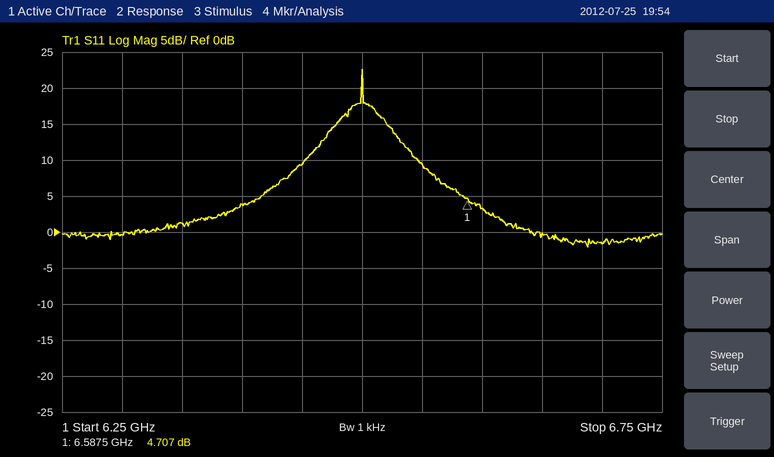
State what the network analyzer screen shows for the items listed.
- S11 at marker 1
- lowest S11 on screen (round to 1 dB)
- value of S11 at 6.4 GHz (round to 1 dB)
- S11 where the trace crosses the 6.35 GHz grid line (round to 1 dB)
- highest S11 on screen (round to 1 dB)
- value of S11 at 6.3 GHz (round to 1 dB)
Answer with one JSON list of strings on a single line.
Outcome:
["4.707 dB", "-2 dB", "4 dB", "1 dB", "23 dB", "0 dB"]
